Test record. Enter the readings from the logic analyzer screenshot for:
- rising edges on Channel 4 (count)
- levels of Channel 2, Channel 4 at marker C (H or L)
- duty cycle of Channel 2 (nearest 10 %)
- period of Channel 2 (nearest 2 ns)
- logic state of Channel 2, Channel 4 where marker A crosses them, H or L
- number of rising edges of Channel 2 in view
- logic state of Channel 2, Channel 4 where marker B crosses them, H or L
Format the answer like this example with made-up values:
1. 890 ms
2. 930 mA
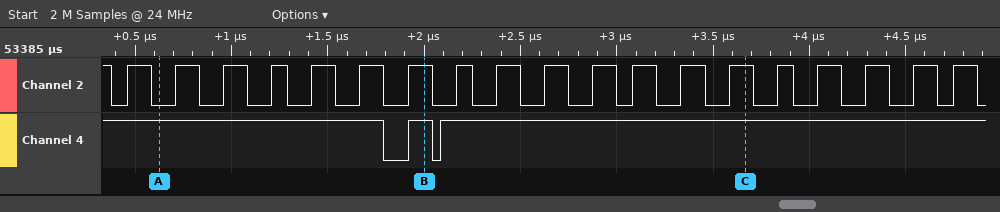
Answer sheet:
1. 2
2. Channel 2=H, Channel 4=H
3. 50 %
4. 238 ns
5. Channel 2=L, Channel 4=H
6. 19
7. Channel 2=H, Channel 4=H
